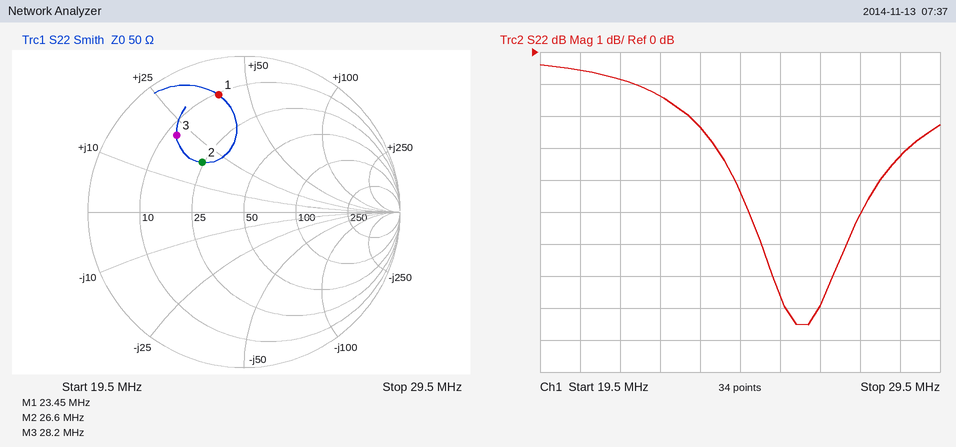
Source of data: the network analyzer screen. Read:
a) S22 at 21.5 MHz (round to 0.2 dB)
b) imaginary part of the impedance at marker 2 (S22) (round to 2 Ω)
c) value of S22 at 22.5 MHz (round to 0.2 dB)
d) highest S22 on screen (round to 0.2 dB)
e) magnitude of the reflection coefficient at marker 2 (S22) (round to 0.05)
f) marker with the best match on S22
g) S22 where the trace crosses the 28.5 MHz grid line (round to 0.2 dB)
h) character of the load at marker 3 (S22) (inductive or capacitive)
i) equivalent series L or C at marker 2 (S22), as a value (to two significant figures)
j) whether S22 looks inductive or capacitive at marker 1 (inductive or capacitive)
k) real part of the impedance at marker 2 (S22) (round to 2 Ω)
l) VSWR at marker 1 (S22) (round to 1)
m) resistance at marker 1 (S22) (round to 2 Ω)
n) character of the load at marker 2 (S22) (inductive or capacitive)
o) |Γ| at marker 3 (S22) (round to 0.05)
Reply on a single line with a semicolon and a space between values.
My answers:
-0.8 dB; +18 Ω; -1.4 dB; -0.4 dB; 0.40; marker 2; -3.2 dB; inductive; 110 nH; inductive; 24 Ω; 8; 10 Ω; inductive; 0.65
